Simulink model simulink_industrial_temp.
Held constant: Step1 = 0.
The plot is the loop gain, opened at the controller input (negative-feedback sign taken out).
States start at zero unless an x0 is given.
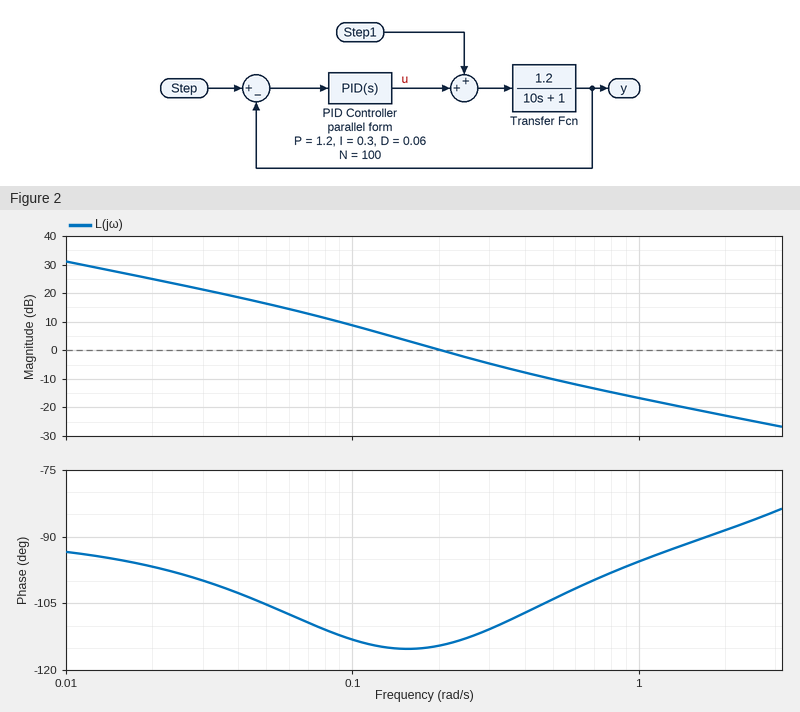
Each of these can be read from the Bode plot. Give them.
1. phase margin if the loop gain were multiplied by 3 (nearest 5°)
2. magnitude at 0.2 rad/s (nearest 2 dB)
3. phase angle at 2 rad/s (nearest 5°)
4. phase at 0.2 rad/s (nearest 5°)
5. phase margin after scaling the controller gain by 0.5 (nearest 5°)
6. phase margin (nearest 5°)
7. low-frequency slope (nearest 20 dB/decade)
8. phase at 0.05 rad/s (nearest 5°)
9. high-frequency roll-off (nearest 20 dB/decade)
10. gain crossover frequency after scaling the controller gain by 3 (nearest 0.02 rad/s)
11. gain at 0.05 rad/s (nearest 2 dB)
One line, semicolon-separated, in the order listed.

75°; 0 dB; -90°; -115°; 65°; 65°; -20 dB/decade; -105°; -20 dB/decade; 0.48 rad/s; 16 dB
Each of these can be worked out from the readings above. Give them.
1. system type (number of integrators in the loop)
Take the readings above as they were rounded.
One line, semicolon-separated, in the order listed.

1
